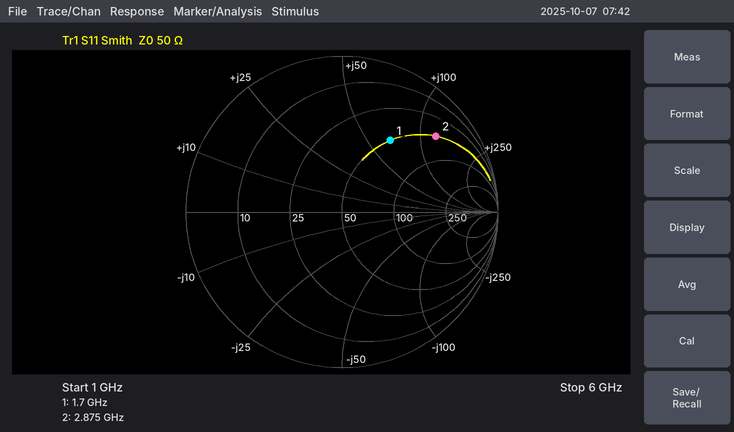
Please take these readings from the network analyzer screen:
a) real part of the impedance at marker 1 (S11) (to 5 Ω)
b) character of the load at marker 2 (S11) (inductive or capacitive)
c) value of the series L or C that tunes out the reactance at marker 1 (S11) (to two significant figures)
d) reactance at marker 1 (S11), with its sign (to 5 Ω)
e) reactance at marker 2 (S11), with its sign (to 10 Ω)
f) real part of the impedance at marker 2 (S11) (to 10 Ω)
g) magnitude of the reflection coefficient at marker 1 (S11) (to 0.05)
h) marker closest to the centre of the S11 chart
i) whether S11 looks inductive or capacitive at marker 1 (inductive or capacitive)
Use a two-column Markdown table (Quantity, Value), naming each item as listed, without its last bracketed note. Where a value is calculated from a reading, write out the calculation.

| Quantity | Value |
|---|---|
| real part of the impedance at marker 1 (S11) | 50 Ω |
| character of the load at marker 2 (S11) | inductive |
| value of the series L or C that tunes out the reactance at marker 1 (S11) | C = 1/(2π × 1.7 GHz × 65 Ω) ≈ 1.4 pF |
| reactance at marker 1 (S11), with its sign | +65 Ω |
| reactance at marker 2 (S11), with its sign | +120 Ω |
| real part of the impedance at marker 2 (S11) | 50 Ω |
| magnitude of the reflection coefficient at marker 1 (S11) | 0.55 |
| marker closest to the centre of the S11 chart | marker 1 |
| whether S11 looks inductive or capacitive at marker 1 | inductive |
